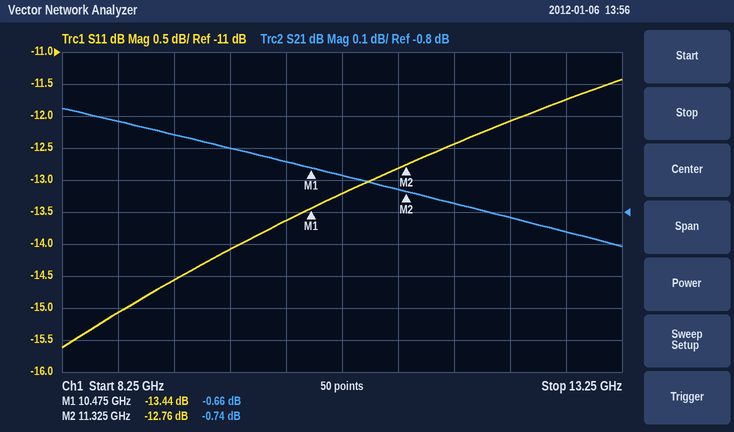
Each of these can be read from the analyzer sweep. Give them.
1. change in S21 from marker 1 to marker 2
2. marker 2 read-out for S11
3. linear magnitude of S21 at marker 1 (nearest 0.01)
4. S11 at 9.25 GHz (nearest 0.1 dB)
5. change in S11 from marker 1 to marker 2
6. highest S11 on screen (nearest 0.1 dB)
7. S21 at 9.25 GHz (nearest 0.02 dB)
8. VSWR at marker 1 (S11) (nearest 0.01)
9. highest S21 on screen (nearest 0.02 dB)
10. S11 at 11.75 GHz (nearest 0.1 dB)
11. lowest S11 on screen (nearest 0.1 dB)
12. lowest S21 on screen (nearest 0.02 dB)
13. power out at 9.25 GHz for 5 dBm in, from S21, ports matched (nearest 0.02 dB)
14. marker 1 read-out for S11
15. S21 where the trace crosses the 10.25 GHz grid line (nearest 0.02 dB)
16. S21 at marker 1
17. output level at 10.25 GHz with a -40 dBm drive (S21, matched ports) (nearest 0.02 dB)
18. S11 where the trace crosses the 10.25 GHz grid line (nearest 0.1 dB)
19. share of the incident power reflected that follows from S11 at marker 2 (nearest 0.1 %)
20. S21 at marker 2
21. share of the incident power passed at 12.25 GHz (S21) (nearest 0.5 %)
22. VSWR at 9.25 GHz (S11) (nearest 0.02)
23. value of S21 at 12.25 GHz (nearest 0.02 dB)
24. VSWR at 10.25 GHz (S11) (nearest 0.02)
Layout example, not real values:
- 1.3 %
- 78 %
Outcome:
- -0.08 dB
- -12.76 dB
- 0.93
- -14.6 dB
- 0.68 dB
- -11.4 dB
- -0.56 dB
- 1.54
- -0.48 dB
- -12.4 dB
- -15.6 dB
- -0.90 dB
- 4.44 dBm
- -13.44 dB
- -0.64 dB
- -0.66 dB
- -40.64 dBm
- -13.6 dB
- 5.3 %
- -0.74 dB
- 83.0 %
- 1.46
- -0.82 dB
- 1.52
